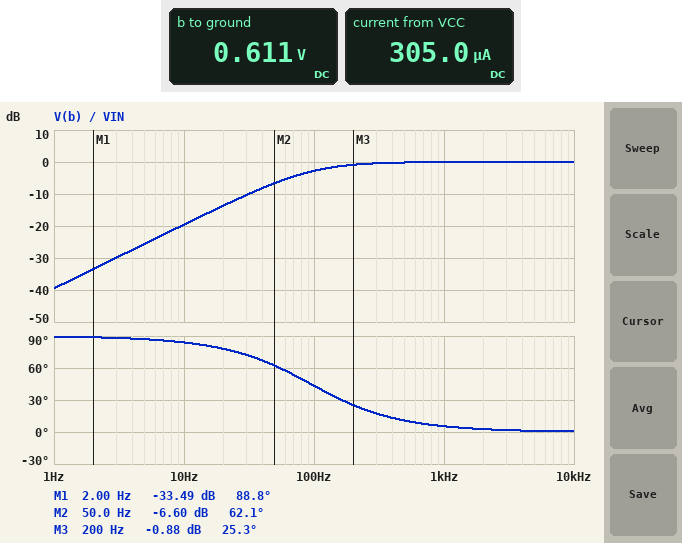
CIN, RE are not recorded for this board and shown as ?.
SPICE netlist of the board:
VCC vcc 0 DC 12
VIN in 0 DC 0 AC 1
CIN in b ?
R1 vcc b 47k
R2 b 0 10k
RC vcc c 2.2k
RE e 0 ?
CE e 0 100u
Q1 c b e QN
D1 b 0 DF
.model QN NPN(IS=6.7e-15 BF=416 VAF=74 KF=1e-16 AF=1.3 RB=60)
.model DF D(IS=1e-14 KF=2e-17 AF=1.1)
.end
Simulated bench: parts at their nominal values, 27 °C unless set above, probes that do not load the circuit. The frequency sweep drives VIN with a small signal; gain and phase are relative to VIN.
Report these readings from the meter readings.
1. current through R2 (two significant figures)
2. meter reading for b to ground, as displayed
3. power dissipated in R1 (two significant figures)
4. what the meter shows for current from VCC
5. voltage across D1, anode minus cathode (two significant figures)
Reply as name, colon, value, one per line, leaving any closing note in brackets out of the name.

current through R2: 61 µA
meter reading for b to ground, as displayed: 0.611 V
power dissipated in R1: 2.8 mW
what the meter shows for current from VCC: 305.0 µA
voltage across D1, anode minus cathode: 610 mV
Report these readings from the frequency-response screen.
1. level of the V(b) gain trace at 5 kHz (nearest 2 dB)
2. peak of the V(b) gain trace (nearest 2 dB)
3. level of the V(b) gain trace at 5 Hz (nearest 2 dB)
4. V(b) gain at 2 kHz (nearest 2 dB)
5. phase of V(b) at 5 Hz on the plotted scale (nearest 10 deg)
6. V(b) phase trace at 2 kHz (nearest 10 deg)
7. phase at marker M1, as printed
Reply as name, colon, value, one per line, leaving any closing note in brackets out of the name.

level of the V(b) gain trace at 5 kHz: 0 dB
peak of the V(b) gain trace: 0 dB
level of the V(b) gain trace at 5 Hz: -26 dB
V(b) gain at 2 kHz: 0 dB
phase of V(b) at 5 Hz on the plotted scale: 90 deg
V(b) phase trace at 2 kHz: 0 deg
phase at marker M1, as printed: 88.8 deg
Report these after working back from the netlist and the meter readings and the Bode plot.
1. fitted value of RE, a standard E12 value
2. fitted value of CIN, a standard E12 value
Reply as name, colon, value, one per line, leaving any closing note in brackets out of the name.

fitted value of RE, a standard E12 value: 330 Ω
fitted value of CIN, a standard E12 value: 12 µF
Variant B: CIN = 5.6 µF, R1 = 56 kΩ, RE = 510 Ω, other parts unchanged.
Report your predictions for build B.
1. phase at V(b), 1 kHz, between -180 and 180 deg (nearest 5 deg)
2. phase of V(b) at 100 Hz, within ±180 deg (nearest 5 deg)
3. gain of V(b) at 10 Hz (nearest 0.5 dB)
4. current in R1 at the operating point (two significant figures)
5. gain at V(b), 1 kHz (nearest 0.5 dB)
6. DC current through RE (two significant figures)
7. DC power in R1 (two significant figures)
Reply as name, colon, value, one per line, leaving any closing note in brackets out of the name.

phase at V(b), 1 kHz, between -180 and 180 deg: 10 deg
phase of V(b) at 100 Hz, within ±180 deg: 60 deg
gain of V(b) at 10 Hz: -24.0 dB
current in R1 at the operating point: 200 µA
gain at V(b), 1 kHz: 0 dB
DC current through RE: 45 µA
DC power in R1: 2.3 mW
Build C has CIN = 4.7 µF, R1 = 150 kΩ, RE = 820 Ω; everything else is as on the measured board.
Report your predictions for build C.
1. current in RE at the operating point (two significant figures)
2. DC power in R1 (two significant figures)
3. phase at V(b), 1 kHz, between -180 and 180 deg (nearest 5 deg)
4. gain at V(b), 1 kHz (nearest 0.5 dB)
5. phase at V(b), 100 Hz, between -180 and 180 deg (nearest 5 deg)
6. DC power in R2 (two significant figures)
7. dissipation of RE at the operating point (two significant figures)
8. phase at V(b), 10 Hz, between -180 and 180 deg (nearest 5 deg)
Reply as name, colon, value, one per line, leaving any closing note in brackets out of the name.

current in RE at the operating point: 11 µA
DC power in R1: 870 µW
phase at V(b), 1 kHz, between -180 and 180 deg: 0 deg
gain at V(b), 1 kHz: 0 dB
phase at V(b), 100 Hz, between -180 and 180 deg: 15 deg
DC power in R2: 31 µW
dissipation of RE at the operating point: 100 nW
phase at V(b), 10 Hz, between -180 and 180 deg: 70 deg
